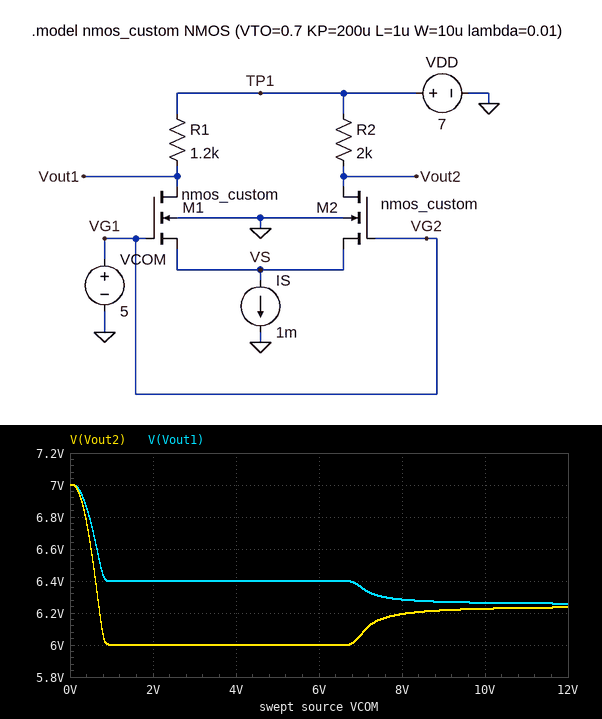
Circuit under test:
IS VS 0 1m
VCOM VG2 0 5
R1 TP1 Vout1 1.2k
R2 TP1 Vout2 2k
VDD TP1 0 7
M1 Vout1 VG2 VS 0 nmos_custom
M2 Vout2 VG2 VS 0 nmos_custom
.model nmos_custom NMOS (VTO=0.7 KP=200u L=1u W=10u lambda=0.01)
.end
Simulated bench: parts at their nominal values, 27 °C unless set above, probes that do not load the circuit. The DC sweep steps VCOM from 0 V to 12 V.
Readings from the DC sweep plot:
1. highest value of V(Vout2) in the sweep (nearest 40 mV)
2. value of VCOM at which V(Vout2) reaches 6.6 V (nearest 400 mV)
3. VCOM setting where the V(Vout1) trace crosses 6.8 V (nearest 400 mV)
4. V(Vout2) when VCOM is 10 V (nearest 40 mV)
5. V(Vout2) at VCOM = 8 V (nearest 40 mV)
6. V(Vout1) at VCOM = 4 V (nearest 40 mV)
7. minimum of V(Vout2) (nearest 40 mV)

7.00 V
400 mV
400 mV
6.24 V
6.20 V
6.40 V
6.00 V
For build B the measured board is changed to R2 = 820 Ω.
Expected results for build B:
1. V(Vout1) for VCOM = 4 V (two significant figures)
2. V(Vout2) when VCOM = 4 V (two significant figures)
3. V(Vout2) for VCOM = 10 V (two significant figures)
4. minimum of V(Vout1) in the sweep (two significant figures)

6.4 V
6.6 V
6.5 V
6.4 V
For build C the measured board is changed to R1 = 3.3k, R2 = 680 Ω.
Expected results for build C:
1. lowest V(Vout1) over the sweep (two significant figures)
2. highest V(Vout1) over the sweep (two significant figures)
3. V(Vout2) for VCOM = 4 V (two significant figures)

5.4 V
7.0 V
6.7 V
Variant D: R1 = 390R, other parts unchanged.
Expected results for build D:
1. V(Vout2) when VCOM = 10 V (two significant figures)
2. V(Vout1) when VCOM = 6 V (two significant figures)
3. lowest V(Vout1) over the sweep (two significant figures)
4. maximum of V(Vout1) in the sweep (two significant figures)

6.6 V
6.8 V
6.7 V
7.0 V
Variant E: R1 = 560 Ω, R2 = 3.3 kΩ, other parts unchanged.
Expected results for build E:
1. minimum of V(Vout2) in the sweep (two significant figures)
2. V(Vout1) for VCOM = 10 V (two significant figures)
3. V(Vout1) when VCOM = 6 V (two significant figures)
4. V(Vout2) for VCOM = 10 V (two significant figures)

5.4 V
6.5 V
6.7 V
6.4 V
